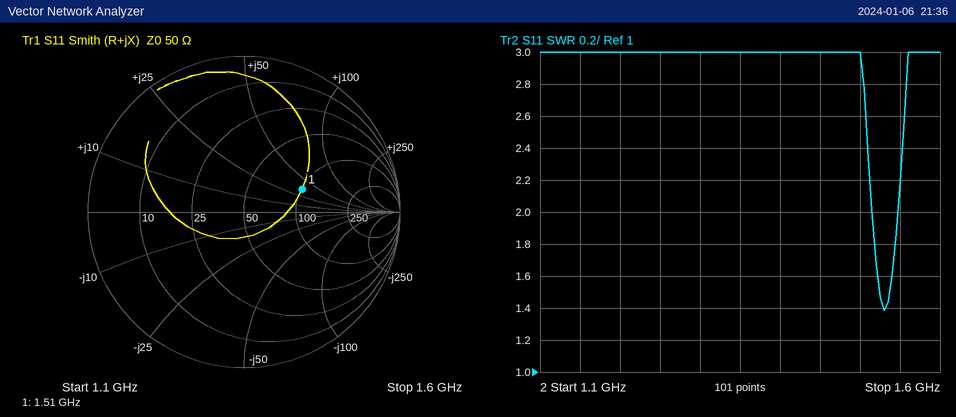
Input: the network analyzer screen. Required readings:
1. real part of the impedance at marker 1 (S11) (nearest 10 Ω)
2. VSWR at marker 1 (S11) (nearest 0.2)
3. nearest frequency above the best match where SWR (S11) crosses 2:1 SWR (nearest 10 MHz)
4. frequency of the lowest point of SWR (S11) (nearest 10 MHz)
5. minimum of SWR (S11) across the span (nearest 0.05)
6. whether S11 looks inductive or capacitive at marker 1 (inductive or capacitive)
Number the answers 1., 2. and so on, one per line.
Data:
1. 100 Ω
2. 2.4
3. 1.55 GHz
4. 1.53 GHz
5. 1.40
6. inductive
